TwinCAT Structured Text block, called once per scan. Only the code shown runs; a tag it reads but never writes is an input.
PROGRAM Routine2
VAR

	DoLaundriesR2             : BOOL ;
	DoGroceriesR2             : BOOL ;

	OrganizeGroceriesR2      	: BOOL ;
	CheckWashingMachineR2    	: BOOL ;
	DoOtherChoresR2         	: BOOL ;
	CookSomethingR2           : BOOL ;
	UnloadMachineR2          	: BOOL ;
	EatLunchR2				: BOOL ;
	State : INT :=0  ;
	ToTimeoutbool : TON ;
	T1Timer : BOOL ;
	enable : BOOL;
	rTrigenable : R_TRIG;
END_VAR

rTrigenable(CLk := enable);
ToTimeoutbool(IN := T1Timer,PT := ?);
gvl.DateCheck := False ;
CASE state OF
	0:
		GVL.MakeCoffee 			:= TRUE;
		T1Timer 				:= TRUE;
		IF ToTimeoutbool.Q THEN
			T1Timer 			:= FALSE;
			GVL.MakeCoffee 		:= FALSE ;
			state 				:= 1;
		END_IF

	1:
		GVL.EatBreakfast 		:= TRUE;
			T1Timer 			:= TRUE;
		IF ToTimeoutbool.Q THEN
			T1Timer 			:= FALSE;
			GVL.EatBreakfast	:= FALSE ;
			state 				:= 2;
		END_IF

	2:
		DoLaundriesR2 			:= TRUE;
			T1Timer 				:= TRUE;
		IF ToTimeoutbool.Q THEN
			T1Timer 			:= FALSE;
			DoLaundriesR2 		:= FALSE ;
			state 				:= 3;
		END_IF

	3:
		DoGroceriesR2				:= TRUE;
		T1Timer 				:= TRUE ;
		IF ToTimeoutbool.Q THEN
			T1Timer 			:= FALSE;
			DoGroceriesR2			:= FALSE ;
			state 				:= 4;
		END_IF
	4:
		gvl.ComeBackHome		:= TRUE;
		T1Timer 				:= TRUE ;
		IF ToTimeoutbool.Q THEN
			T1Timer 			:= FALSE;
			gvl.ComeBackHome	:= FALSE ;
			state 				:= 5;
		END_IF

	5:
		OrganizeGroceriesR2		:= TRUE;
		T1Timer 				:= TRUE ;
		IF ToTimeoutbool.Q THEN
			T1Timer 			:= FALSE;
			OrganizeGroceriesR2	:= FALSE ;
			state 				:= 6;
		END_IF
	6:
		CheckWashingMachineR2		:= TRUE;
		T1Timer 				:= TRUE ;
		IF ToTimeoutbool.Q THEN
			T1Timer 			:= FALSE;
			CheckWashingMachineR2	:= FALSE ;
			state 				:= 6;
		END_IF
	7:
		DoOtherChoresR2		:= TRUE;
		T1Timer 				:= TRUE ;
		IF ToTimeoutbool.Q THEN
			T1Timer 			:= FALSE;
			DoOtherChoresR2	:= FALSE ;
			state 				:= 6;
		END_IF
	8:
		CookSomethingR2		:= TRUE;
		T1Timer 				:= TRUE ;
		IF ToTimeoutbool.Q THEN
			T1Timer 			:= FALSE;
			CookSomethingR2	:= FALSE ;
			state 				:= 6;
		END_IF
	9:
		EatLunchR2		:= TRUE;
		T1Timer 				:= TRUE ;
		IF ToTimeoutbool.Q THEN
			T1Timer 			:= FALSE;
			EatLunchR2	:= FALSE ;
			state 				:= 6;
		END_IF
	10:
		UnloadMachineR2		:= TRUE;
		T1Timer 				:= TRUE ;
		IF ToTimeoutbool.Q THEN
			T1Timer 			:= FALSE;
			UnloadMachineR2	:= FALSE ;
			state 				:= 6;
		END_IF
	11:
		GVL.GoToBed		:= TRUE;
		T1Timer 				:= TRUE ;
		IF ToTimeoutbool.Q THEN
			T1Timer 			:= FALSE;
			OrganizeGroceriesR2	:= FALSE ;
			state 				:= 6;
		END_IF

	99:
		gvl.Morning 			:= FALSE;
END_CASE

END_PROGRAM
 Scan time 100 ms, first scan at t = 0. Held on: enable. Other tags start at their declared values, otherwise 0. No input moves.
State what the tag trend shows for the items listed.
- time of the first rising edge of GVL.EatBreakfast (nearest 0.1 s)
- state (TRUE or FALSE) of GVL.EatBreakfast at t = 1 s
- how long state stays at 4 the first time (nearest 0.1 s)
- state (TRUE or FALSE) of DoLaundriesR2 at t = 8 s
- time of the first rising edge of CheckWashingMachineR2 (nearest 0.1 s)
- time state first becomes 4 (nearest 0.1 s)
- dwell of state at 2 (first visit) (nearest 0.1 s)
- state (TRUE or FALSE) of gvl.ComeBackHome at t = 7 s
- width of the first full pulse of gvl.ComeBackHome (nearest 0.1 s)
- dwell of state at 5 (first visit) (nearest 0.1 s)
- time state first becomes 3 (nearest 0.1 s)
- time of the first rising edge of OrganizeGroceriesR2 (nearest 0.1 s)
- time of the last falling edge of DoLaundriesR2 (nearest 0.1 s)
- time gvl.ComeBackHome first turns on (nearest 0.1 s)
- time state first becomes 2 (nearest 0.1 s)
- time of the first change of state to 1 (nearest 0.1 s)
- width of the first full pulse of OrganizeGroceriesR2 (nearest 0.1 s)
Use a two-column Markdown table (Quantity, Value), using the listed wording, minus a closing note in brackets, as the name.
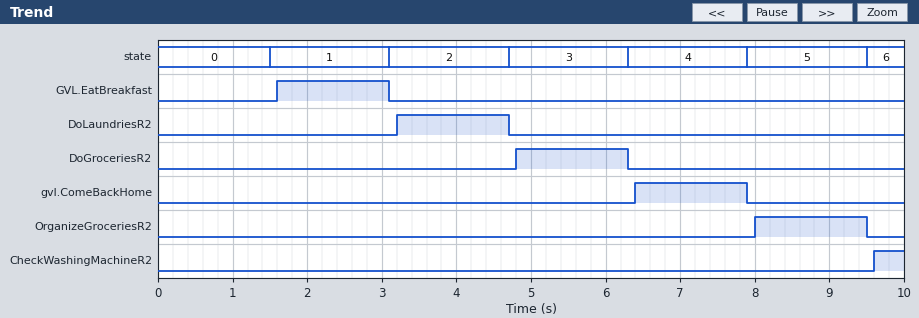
| Quantity | Value |
|---|---|
| time of the first rising edge of GVL.EatBreakfast | 1.6 s |
| state (TRUE or FALSE) of GVL.EatBreakfast at t = 1 s | FALSE |
| how long state stays at 4 the first time | 1.6 s |
| state (TRUE or FALSE) of DoLaundriesR2 at t = 8 s | FALSE |
| time of the first rising edge of CheckWashingMachineR2 | 9.6 s |
| time state first becomes 4 | 6.3 s |
| dwell of state at 2 (first visit) | 1.6 s |
| state (TRUE or FALSE) of gvl.ComeBackHome at t = 7 s | TRUE |
| width of the first full pulse of gvl.ComeBackHome | 1.5 s |
| dwell of state at 5 (first visit) | 1.6 s |
| time state first becomes 3 | 4.7 s |
| time of the first rising edge of OrganizeGroceriesR2 | 8.0 s |
| time of the last falling edge of DoLaundriesR2 | 4.7 s |
| time gvl.ComeBackHome first turns on | 6.4 s |
| time state first becomes 2 | 3.1 s |
| time of the first change of state to 1 | 1.5 s |
| width of the first full pulse of OrganizeGroceriesR2 | 1.5 s |
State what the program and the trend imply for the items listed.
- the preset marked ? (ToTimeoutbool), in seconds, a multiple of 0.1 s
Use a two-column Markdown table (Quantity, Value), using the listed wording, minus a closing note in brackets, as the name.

| Quantity | Value |
|---|---|
| the preset marked ? (ToTimeoutbool), in seconds, a multiple of 0.1 s | 1.4 s |
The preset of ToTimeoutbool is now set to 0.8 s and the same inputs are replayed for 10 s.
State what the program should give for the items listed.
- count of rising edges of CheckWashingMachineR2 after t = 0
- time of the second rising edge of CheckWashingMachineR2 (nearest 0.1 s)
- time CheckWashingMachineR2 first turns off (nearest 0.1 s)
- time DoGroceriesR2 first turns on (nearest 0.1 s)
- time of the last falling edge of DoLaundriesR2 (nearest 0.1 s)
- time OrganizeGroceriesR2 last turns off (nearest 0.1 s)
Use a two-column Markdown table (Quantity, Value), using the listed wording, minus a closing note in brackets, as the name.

| Quantity | Value |
|---|---|
| count of rising edges of CheckWashingMachineR2 after t = 0 | 4 |
| time of the second rising edge of CheckWashingMachineR2 | 7.0 s |
| time CheckWashingMachineR2 first turns off | 6.9 s |
| time DoGroceriesR2 first turns on | 3.0 s |
| time of the last falling edge of DoLaundriesR2 | 2.9 s |
| time OrganizeGroceriesR2 last turns off | 5.9 s |
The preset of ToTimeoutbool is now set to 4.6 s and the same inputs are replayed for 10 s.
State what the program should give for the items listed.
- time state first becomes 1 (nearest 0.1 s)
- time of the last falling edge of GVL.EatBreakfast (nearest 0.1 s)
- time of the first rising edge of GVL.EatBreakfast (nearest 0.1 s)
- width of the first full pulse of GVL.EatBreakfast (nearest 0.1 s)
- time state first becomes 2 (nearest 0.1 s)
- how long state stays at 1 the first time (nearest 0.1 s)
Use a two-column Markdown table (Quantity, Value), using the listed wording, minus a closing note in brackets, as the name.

| Quantity | Value |
|---|---|
| time state first becomes 1 | 4.7 s |
| time of the last falling edge of GVL.EatBreakfast | 9.5 s |
| time of the first rising edge of GVL.EatBreakfast | 4.8 s |
| width of the first full pulse of GVL.EatBreakfast | 4.7 s |
| time state first becomes 2 | 9.5 s |
| how long state stays at 1 the first time | 4.8 s |
